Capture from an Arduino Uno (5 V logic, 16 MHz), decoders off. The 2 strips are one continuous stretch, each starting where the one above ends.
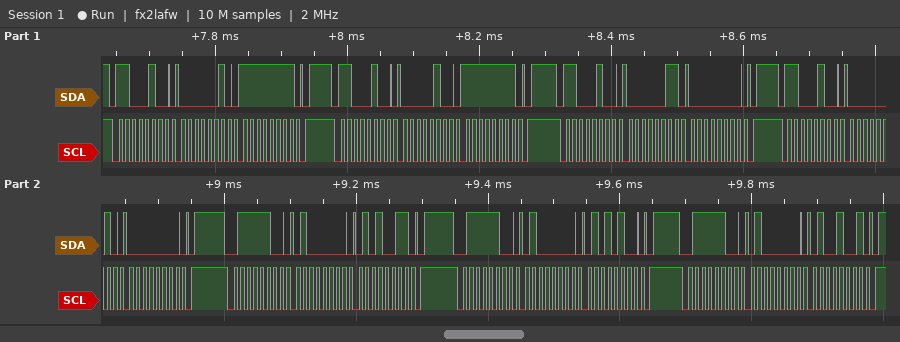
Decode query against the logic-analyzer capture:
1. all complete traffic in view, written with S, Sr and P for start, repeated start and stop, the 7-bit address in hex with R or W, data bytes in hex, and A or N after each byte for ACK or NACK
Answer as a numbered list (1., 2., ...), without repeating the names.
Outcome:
1. S 62W A 02 A FF A P S 62W A 04 A FF A P S 62W A 03 A 00 A P S 62W A 02 A 00 A P S 3EW A 40 A 53 A P S 3EW A 40 A 54 A P S 3EW A 40 A 49 A P
